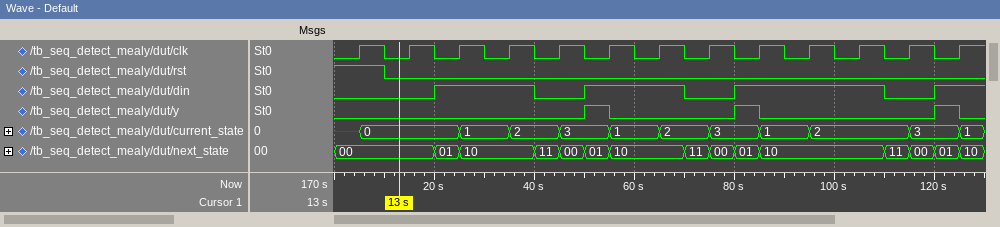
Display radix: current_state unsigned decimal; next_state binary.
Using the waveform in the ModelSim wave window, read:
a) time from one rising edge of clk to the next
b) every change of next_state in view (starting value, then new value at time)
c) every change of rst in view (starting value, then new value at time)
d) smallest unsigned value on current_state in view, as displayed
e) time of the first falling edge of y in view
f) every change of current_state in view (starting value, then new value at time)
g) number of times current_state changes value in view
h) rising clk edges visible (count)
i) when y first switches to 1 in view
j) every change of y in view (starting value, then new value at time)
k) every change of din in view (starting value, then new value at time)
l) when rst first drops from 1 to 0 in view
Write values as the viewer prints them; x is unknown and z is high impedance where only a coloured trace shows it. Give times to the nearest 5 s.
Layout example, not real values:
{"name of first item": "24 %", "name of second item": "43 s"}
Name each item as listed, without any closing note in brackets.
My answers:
{"time from one rising edge of clk to the next": "10 s", "every change of next_state in view": "00, 01 at 20 s, 10 at 25 s, 11 at 40 s, 00 at 45 s, 01 at 50 s, 10 at 55 s, 11 at 70 s, 00 at 75 s, 01 at 80 s, 10 at 85 s, 11 at 110 s, 00 at 115 s, 01 at 120 s, 10 at 125 s", "every change of rst in view": "1, 0 at 10 s", "smallest unsigned value on current_state in view, as displayed": "0", "time of the first falling edge of y in view": "55 s", "every change of current_state in view": "x, 0 at 5 s, 1 at 25 s, 2 at 35 s, 3 at 45 s, 1 at 55 s, 2 at 65 s, 3 at 75 s, 1 at 85 s, 2 at 95 s, 3 at 115 s, 1 at 125 s", "number of times current_state changes value in view": "11", "rising clk edges visible": "13", "when y first switches to 1 in view": "50 s", "every change of y in view": "0, 1 at 50 s, 0 at 55 s, 1 at 80 s, 0 at 85 s, 1 at 120 s, 0 at 125 s", "every change of din in view": "0, 1 at 20 s, 0 at 40 s, 1 at 50 s, 0 at 70 s, 1 at 80 s, 0 at 110 s, 1 at 120 s", "when rst first drops from 1 to 0 in view": "10 s"}
